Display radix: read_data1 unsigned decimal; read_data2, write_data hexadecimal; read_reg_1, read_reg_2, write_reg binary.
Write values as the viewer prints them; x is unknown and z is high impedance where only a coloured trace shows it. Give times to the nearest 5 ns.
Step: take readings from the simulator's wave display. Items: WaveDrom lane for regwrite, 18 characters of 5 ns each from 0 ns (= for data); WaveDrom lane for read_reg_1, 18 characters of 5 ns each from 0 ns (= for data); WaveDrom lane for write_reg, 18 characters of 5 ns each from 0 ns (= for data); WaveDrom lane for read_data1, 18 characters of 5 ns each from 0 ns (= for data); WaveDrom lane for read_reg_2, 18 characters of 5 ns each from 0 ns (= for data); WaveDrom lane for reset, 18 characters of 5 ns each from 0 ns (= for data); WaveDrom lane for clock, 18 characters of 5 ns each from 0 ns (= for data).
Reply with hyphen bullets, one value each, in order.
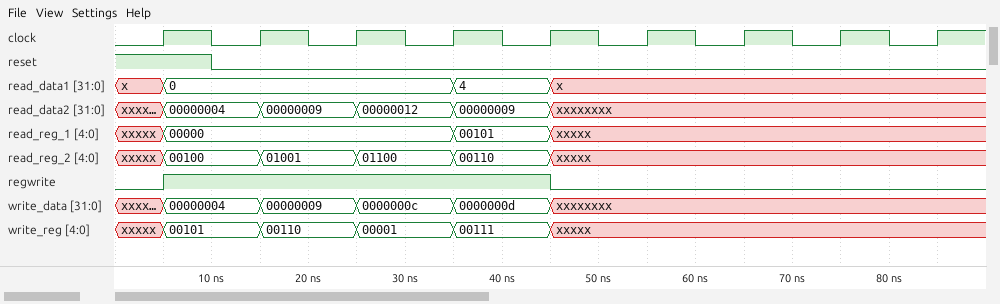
- {name: 'regwrite', wave: '01.......0........'}
- {name: 'read_reg_1', wave: 'x=.....=.x........', data: '00000 00101'}
- {name: 'write_reg', wave: 'x=.=.=.=.x........', data: '00101 00110 00001 00111'}
- {name: 'read_data1', wave: 'x=.....=.x........', data: '0 4'}
- {name: 'read_reg_2', wave: 'x=.=.=.=.x........', data: '00100 01001 01100 00110'}
- {name: 'reset', wave: '1.0...............'}
- {name: 'clock', wave: '010101010101010101'}
